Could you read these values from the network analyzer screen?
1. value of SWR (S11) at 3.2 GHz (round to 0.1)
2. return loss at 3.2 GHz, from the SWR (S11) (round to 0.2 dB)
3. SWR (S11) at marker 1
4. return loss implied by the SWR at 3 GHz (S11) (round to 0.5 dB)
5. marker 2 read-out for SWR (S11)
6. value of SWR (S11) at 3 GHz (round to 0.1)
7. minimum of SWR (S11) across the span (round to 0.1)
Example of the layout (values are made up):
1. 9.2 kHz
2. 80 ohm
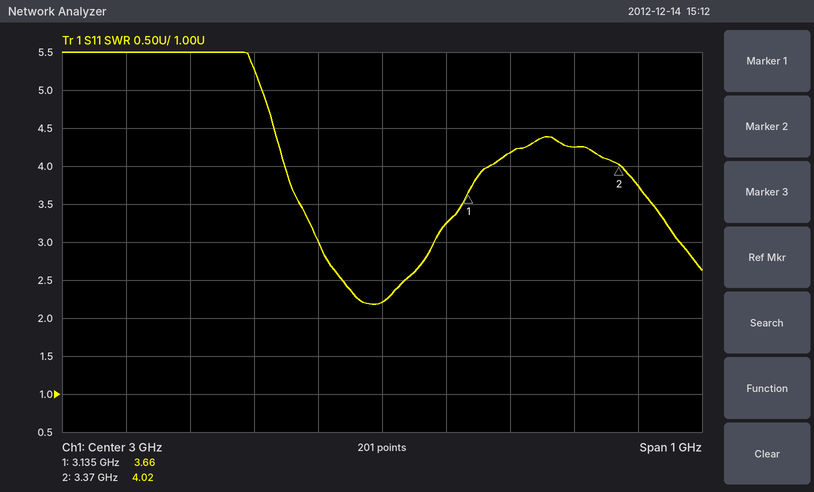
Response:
1. 4.2
2. 4.2 dB
3. 3.66
4. 8.5 dB
5. 4.02
6. 2.2
7. 2.2
